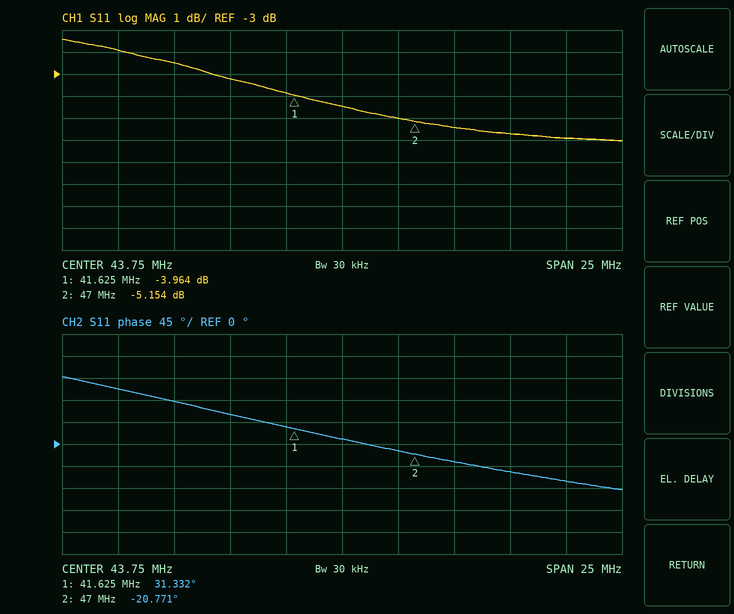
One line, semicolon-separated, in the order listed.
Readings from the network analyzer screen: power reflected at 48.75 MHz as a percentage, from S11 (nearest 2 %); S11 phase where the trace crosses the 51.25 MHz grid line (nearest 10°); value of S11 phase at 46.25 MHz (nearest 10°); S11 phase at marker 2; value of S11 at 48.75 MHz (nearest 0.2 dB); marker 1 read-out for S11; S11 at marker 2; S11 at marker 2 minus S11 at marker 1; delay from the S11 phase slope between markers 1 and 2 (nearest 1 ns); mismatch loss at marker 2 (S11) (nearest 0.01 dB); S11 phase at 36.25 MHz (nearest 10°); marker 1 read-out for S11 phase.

28 %; -60°; -10°; -20.771°; -5.4 dB; -3.964 dB; -5.154 dB; -1.190 dB; 27 ns; 1.58 dB; 90°; 31.332°
